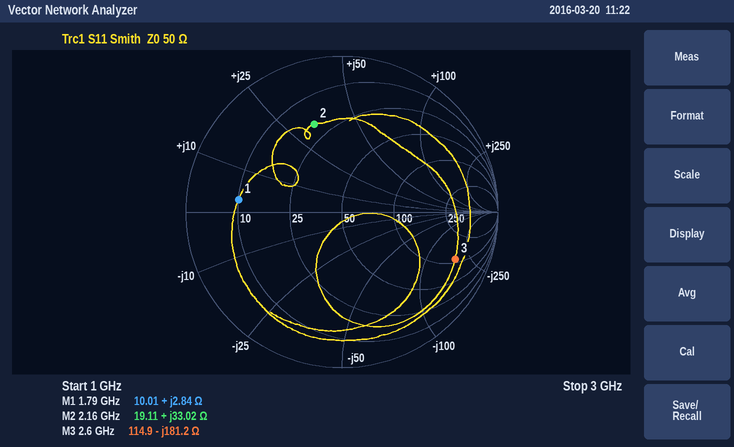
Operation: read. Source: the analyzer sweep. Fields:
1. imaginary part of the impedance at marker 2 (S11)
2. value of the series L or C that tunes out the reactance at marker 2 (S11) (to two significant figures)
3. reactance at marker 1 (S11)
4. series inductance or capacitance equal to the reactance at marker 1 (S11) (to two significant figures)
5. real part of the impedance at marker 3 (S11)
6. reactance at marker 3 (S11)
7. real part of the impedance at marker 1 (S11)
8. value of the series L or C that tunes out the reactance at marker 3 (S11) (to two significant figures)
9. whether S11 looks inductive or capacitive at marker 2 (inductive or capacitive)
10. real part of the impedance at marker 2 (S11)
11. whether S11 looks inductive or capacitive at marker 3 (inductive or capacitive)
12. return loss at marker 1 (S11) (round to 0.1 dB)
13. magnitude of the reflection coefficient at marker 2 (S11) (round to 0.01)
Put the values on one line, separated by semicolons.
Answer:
+33.02 Ω; 2.2 pF; +2.84 Ω; 250 pH; 114.9 Ω; -181.2 Ω; 10.01 Ω; 11 nH; inductive; 19.11 Ω; capacitive; 3.5 dB; 0.59
